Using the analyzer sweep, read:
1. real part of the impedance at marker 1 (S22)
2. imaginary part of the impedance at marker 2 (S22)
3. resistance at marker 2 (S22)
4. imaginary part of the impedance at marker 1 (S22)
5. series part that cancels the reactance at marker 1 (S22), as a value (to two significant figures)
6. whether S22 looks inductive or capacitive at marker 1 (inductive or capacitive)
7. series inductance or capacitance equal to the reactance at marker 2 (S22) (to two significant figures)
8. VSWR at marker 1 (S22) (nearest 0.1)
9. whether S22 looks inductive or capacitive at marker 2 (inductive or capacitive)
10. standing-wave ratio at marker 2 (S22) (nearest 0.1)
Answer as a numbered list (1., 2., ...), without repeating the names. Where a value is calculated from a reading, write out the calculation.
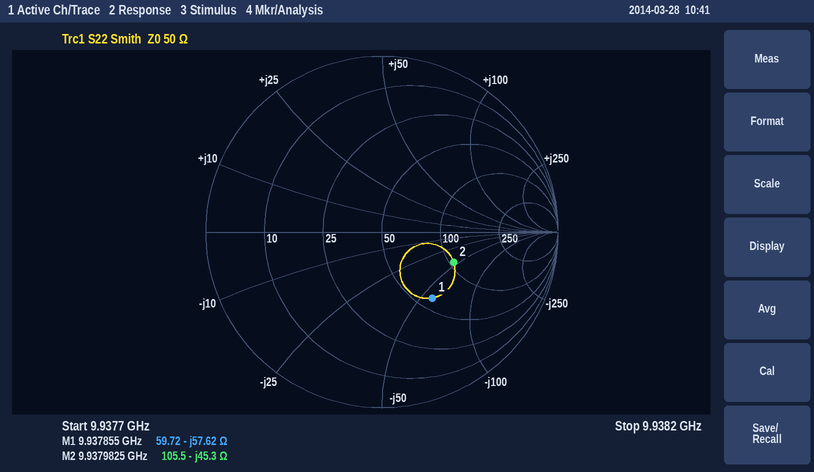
1. 59.72 Ω
2. -45.3 Ω
3. 105.5 Ω
4. -57.62 Ω
5. L = 57.62 Ω/(2π × 9.937855 GHz) ≈ 923 pH, so 920 pH to two significant figures
6. capacitive
7. C = 1/(2π × 9.9379825 GHz × 45.3 Ω) ≈ 354 fF, so 350 fF to two significant figures
8. 2.8
9. capacitive
10. 2.6
